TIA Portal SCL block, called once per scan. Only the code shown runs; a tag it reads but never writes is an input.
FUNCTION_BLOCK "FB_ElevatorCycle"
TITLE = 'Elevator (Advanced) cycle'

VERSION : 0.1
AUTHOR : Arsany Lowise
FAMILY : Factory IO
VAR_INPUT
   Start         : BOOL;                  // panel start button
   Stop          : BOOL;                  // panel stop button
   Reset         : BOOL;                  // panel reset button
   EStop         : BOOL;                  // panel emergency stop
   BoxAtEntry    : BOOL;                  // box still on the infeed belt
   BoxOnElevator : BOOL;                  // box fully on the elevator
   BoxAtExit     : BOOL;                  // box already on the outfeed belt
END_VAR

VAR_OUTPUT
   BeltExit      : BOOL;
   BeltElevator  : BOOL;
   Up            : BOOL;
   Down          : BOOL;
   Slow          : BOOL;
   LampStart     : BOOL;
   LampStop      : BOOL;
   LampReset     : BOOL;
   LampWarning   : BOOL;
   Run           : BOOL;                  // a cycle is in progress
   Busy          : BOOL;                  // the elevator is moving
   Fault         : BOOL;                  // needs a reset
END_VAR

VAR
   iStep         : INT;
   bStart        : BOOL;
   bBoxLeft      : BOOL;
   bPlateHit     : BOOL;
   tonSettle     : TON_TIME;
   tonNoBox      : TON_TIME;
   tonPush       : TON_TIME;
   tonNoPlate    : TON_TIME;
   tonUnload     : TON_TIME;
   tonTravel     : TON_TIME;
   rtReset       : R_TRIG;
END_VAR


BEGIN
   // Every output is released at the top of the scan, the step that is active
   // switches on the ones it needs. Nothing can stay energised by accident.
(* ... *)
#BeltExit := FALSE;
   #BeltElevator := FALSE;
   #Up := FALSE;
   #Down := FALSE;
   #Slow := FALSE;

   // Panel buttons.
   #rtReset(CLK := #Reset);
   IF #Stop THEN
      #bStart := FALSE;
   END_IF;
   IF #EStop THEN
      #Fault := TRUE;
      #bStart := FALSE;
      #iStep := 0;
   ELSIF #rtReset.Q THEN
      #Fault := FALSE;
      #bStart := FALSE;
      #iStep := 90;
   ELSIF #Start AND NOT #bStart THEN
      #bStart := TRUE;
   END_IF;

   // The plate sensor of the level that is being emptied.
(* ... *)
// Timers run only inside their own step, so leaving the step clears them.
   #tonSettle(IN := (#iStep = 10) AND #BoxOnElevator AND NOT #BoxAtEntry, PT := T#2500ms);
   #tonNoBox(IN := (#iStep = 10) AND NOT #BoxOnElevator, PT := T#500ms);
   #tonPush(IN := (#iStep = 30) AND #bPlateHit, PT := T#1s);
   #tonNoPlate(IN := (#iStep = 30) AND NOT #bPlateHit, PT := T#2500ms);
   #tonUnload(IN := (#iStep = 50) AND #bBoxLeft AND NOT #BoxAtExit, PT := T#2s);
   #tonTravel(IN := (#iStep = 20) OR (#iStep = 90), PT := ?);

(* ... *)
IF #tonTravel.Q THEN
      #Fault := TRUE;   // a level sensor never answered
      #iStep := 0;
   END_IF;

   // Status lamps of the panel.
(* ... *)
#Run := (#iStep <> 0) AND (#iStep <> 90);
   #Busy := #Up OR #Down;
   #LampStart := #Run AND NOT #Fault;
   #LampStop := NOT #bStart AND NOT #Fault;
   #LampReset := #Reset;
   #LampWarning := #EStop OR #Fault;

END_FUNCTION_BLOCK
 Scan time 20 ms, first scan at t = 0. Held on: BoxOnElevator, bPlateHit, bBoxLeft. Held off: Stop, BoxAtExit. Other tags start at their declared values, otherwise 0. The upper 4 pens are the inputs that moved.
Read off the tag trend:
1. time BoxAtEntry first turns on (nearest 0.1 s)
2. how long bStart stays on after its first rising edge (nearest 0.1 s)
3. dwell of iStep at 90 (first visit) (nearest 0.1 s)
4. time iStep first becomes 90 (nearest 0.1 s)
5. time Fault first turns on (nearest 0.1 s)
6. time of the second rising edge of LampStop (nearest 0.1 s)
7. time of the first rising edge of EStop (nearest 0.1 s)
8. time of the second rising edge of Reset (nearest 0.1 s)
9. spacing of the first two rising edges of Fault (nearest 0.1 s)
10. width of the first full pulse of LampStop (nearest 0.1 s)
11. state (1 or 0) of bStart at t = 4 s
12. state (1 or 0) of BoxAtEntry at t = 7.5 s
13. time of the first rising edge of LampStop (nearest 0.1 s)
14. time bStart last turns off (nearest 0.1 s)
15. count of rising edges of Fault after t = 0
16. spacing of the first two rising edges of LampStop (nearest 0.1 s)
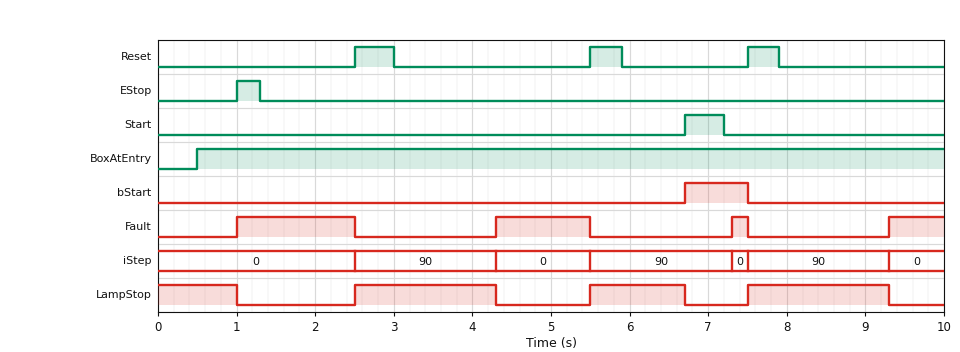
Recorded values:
0.5 s
0.8 s
1.8 s
2.5 s
1.0 s
5.5 s
1.0 s
5.5 s
3.3 s
1.8 s
0
1
2.5 s
7.5 s
4
3.0 s
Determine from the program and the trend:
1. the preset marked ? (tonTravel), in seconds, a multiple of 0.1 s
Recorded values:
1.8 s
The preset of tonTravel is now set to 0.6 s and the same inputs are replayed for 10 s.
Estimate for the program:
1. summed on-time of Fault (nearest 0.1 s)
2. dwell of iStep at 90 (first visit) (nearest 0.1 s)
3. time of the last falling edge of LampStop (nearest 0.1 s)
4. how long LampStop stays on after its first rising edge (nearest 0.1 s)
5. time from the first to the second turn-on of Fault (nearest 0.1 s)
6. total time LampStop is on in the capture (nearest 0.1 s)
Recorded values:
7.2 s
0.6 s
8.1 s
0.6 s
2.1 s
2.8 s
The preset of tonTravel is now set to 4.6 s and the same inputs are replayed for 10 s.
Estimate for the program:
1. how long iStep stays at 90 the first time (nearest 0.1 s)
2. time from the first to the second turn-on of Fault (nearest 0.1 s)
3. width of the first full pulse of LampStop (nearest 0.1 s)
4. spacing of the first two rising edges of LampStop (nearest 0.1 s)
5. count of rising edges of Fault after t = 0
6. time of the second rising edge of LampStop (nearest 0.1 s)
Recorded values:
4.6 s
6.1 s
4.2 s
5.0 s
2
7.5 s
